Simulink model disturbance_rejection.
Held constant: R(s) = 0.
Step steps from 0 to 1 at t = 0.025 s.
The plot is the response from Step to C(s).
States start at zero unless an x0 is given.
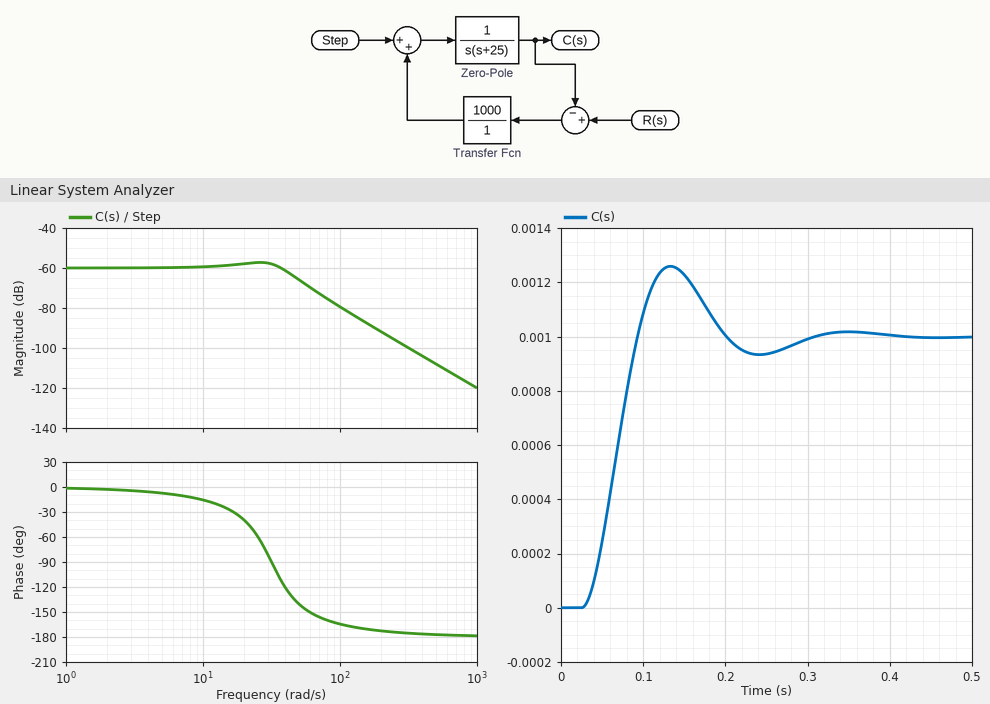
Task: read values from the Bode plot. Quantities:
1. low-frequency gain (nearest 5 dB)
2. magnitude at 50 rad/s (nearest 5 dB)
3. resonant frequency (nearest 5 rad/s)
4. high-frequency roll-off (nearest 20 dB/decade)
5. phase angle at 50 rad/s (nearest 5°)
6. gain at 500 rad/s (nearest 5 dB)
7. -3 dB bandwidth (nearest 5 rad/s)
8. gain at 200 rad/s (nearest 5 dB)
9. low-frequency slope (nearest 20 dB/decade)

-60 dB
-65 dB
25 rad/s
-40 dB/decade
-140°
-110 dB
45 rad/s
-90 dB
0 dB/decade
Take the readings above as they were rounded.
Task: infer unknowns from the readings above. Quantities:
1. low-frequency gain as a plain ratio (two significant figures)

0.0010
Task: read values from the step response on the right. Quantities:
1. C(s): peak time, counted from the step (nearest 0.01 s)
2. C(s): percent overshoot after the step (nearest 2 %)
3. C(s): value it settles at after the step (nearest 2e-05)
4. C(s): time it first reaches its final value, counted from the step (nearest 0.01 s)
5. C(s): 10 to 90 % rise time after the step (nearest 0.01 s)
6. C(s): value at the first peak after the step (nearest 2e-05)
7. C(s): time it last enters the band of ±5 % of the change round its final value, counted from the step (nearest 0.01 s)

0.11 s
26 %
0.00100
0.07 s
0.05 s
0.00126
0.24 s
